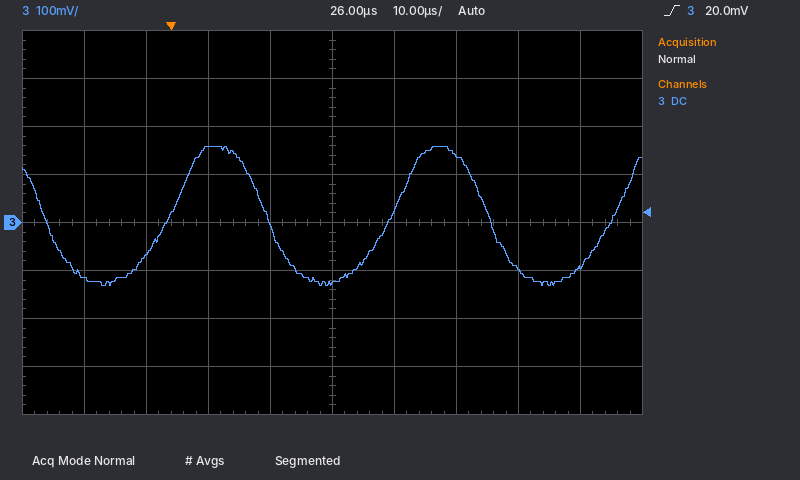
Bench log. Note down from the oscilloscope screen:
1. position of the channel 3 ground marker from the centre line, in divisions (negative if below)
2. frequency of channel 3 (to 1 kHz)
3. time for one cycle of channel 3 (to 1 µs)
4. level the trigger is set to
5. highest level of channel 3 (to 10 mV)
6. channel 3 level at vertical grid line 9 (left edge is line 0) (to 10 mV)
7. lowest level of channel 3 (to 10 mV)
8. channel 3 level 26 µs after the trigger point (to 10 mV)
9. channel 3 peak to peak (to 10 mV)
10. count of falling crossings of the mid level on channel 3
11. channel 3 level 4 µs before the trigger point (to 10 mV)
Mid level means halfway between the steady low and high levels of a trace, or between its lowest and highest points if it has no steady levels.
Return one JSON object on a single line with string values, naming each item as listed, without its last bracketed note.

{"position of the channel 3 ground marker from the centre line, in divisions": "0.0 div", "frequency of channel 3": "28 kHz", "time for one cycle of channel 3": "36 µs", "level the trigger is set to": "20.0 mV", "highest level of channel 3": "160 mV", "channel 3 level at vertical grid line 9 (left edge is line 0)": "-90 mV", "lowest level of channel 3": "-130 mV", "channel 3 level 26 µs after the trigger point": "-130 mV", "channel 3 peak to peak": "290 mV", "count of falling crossings of the mid level on channel 3": "3", "channel 3 level 4 µs before the trigger point": "-70 mV"}
